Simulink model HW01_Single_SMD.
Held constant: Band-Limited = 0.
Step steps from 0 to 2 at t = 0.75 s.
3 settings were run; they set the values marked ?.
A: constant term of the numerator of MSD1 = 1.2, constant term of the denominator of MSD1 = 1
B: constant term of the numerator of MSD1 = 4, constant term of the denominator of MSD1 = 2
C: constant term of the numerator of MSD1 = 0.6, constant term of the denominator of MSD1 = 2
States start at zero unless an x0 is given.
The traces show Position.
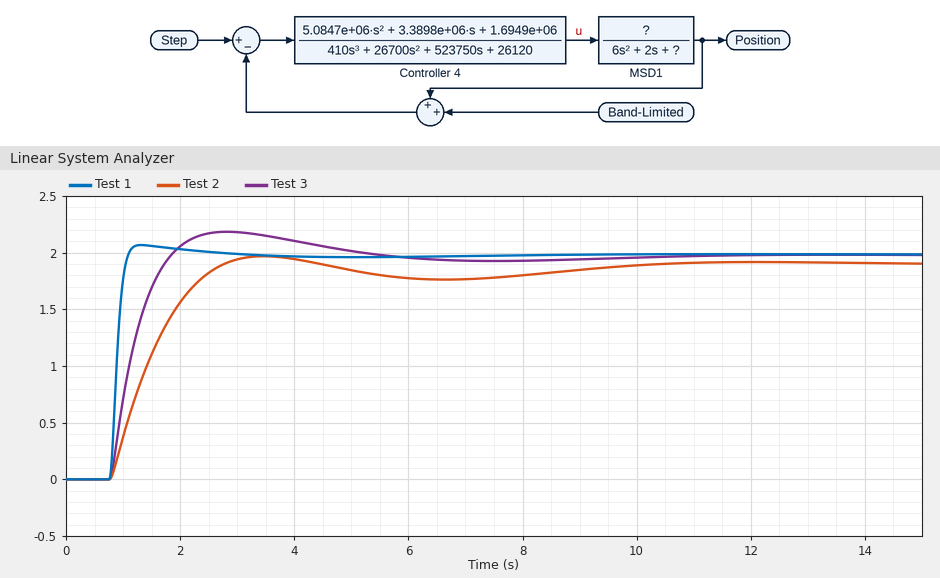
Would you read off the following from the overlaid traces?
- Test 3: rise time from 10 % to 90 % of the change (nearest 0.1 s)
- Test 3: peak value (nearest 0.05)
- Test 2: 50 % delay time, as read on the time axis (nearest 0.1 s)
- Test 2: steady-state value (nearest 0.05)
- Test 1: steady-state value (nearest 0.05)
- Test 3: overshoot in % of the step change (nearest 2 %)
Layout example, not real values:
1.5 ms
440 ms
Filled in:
0.7 s
2.20
1.4 s
1.90
2.00
10 %
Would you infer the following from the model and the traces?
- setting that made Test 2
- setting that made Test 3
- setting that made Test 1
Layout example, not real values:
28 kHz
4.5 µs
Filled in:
C
A
B
